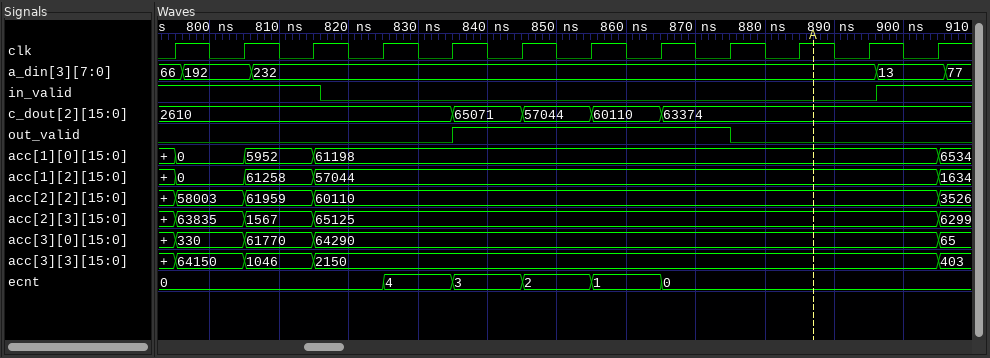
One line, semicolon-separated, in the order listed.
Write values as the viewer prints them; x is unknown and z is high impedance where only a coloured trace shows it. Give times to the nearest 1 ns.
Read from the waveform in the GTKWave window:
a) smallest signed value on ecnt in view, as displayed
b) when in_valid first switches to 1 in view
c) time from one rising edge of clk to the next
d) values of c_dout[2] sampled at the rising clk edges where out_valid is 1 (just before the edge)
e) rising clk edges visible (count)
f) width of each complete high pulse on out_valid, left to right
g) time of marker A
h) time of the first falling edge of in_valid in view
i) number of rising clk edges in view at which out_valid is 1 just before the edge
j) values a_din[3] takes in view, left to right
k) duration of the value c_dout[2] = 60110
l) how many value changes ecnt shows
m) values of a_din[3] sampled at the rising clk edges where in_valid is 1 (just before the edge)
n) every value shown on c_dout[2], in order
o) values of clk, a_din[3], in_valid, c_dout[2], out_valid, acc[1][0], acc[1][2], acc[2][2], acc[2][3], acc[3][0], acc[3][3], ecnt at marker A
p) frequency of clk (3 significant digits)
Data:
0; 896 ns; 10 ns; 65071, 57044, 60110, 63374; 12; 40 ns; 887 ns; 816 ns; 4; 66, 192, 232, 13, 77; 10 ns; 5; 66, 192, 232, 13; 2610, 65071, 57044, 60110, 63374; clk=1, a_din[3]=232, in_valid=0, c_dout[2]=63374, out_valid=0, acc[1][0]=61198, acc[1][2]=57044, acc[2][2]=60110, acc[2][3]=65125, acc[3][0]=64290, acc[3][3]=2150, ecnt=0; 100 MHz
